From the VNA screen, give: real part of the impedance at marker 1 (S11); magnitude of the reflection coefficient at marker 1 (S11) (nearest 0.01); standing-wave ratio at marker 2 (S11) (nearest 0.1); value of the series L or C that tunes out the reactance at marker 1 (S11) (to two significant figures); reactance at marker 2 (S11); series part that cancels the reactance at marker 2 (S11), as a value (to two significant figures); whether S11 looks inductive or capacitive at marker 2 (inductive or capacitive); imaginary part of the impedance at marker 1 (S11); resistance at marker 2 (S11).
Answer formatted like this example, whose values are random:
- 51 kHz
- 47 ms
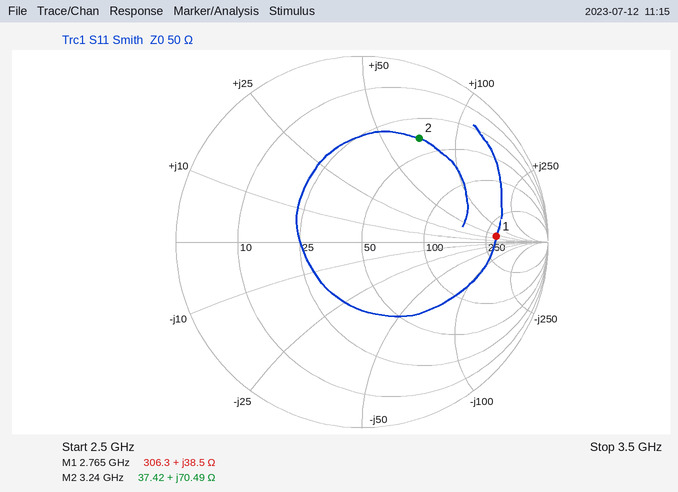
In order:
- 306.3 Ω
- 0.72
- 4.5
- 1.5 pF
- +70.49 Ω
- 700 fF
- inductive
- +38.5 Ω
- 37.42 Ω
